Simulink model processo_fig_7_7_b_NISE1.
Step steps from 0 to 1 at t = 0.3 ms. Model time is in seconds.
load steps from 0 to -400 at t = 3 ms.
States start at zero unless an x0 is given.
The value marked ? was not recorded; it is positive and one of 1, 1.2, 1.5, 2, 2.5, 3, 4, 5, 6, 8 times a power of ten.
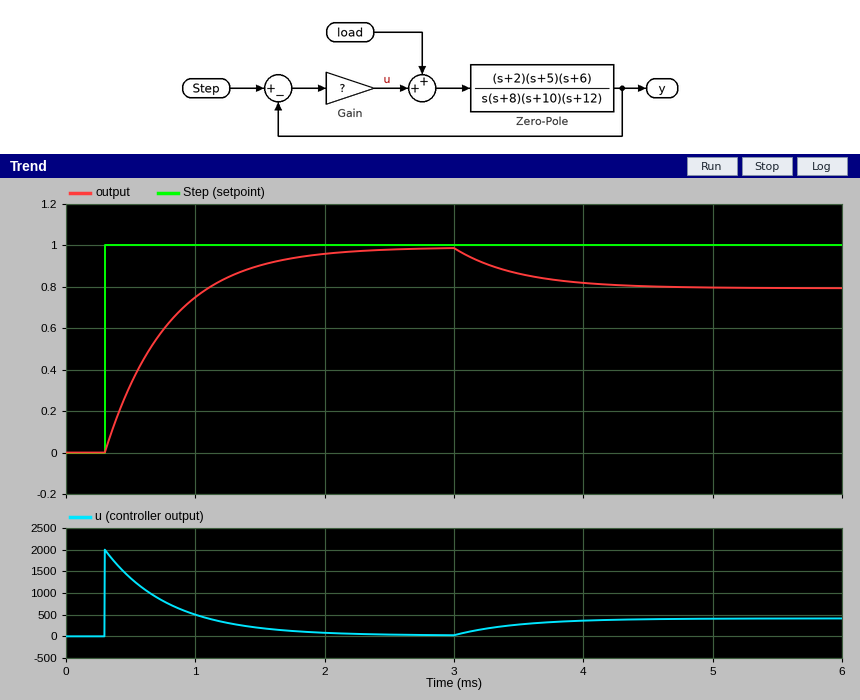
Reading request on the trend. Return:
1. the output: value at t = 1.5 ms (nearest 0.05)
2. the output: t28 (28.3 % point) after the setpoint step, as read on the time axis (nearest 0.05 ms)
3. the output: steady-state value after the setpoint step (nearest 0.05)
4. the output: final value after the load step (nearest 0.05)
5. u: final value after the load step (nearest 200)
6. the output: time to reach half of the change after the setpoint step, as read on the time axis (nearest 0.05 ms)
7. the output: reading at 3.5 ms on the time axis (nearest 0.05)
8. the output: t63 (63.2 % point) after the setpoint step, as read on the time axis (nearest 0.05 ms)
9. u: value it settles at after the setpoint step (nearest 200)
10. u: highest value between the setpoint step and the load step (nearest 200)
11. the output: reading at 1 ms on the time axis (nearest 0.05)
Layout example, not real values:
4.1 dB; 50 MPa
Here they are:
0.90; 0.45 ms; 1.00; 0.80; 400; 0.65 ms; 0.85; 0.80 ms; 0; 2000; 0.75
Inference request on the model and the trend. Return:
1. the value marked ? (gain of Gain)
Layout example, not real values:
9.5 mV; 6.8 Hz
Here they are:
2000
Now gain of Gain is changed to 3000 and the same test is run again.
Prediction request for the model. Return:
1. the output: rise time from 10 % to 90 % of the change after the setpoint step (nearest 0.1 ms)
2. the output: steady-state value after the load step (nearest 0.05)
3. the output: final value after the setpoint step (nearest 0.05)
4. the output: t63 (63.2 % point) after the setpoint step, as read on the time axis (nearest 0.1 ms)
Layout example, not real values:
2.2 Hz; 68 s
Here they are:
0.7 ms; 0.85; 1.00; 0.6 ms
